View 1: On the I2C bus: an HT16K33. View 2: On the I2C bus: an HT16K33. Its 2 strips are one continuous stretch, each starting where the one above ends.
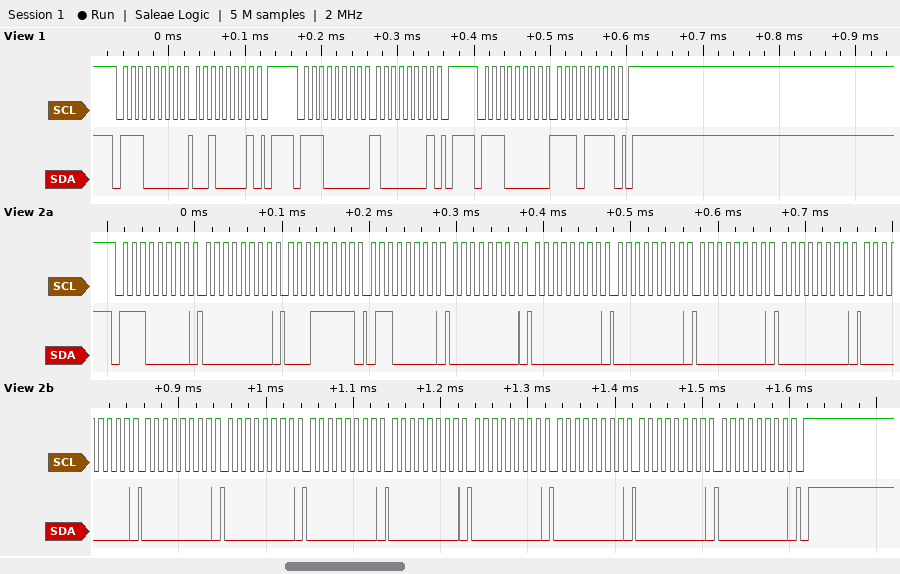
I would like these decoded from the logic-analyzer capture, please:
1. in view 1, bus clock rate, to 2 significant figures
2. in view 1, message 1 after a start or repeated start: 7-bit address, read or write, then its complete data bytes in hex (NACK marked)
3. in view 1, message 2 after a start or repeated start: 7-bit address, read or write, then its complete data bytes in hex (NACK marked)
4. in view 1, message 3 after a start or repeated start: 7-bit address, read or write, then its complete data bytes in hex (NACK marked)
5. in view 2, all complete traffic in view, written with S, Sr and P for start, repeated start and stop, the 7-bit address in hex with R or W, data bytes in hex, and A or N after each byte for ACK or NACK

100 kHz
0x70 write: 21
0x70 write: 81
0x70 write: EF
S 70W A 00 A 1F A 60 A 00 A 00 A 00 A 00 A 00 A 00 A 00 A 00 A 00 A 00 A 00 A 00 A 00 A 00 A P
